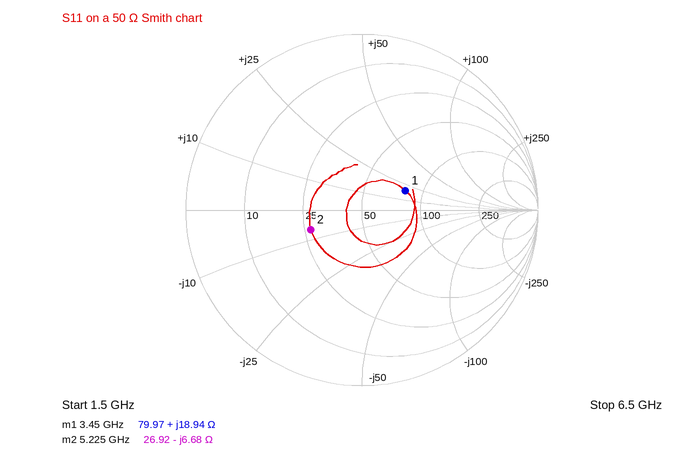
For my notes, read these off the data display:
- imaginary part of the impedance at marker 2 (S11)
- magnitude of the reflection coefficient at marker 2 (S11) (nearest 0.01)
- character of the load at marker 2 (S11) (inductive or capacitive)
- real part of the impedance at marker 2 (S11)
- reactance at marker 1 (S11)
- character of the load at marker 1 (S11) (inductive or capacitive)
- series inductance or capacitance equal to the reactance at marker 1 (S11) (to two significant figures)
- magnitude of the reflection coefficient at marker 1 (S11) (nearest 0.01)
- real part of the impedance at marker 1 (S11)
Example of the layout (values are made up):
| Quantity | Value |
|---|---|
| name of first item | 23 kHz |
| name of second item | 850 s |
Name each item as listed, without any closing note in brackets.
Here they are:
| Quantity | Value |
|---|---|
| imaginary part of the impedance at marker 2 | -6.68 Ω |
| magnitude of the reflection coefficient at marker 2 (S11) | 0.31 |
| character of the load at marker 2 (S11) | capacitive |
| real part of the impedance at marker 2 | 26.92 Ω |
| reactance at marker 1 | +18.94 Ω |
| character of the load at marker 1 (S11) | inductive |
| series inductance or capacitance equal to the reactance at marker 1 (S11) | 870 pH |
| magnitude of the reflection coefficient at marker 1 (S11) | 0.27 |
| real part of the impedance at marker 1 | 79.97 Ω |
